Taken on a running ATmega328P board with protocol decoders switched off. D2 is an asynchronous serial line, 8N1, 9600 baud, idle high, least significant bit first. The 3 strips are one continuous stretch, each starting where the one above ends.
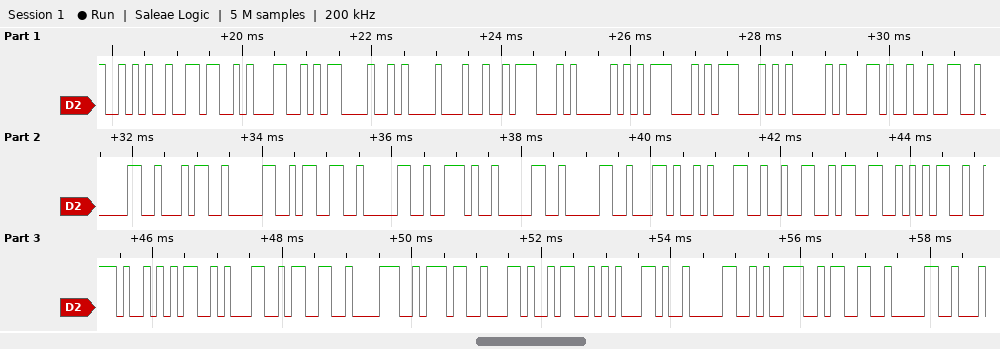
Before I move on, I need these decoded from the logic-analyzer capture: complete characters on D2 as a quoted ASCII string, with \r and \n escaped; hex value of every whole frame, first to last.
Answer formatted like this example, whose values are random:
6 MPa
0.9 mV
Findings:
"*61\r\n$GPGGA,204030.00,1235.51387,S,0930"
2A 36 31 0D 0A 24 47 50 47 47 41 2C 32 30 34 30 33 30 2E 30 30 2C 31 32 33 35 2E 35 31 33 38 37 2C 53 2C 30 39 33 30
